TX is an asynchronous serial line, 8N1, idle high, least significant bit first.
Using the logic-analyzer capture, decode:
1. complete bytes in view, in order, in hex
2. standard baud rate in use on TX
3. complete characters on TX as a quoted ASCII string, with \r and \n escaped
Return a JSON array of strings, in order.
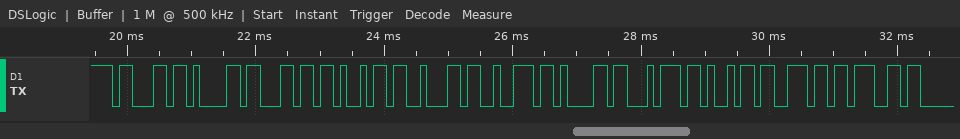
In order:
["0x63 0x61 0x6C 0x69 0x62 0x72 0x61 0x74 0x69 0x6E 0x67", "9600 baud", "\"calibrating\""]
